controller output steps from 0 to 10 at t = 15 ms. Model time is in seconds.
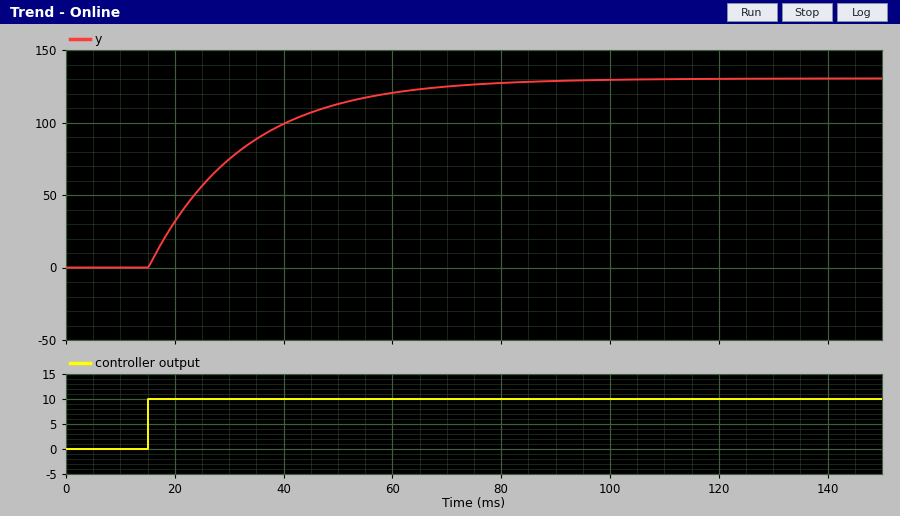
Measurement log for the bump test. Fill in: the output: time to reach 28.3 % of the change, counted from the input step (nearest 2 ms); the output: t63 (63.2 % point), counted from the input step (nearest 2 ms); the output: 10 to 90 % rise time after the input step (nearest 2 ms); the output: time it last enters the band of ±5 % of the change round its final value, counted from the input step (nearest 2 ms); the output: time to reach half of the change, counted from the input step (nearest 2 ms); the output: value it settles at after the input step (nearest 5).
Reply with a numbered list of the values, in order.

1. 6 ms
2. 18 ms
3. 38 ms
4. 52 ms
5. 12 ms
6. 130
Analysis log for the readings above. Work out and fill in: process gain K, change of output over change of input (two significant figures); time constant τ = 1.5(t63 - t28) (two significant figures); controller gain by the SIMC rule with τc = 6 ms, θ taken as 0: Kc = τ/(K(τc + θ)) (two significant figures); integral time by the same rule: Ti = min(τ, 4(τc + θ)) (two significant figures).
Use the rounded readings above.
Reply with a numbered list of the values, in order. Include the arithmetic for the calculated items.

1. (130 - 0) / 10 = 13
2. 1.5 × (18 - 6) = 18 ms
3. 18 / (13 × (6 + 0)) = 0.23
4. min(18, 4 × (6 + 0)) = 18 ms
